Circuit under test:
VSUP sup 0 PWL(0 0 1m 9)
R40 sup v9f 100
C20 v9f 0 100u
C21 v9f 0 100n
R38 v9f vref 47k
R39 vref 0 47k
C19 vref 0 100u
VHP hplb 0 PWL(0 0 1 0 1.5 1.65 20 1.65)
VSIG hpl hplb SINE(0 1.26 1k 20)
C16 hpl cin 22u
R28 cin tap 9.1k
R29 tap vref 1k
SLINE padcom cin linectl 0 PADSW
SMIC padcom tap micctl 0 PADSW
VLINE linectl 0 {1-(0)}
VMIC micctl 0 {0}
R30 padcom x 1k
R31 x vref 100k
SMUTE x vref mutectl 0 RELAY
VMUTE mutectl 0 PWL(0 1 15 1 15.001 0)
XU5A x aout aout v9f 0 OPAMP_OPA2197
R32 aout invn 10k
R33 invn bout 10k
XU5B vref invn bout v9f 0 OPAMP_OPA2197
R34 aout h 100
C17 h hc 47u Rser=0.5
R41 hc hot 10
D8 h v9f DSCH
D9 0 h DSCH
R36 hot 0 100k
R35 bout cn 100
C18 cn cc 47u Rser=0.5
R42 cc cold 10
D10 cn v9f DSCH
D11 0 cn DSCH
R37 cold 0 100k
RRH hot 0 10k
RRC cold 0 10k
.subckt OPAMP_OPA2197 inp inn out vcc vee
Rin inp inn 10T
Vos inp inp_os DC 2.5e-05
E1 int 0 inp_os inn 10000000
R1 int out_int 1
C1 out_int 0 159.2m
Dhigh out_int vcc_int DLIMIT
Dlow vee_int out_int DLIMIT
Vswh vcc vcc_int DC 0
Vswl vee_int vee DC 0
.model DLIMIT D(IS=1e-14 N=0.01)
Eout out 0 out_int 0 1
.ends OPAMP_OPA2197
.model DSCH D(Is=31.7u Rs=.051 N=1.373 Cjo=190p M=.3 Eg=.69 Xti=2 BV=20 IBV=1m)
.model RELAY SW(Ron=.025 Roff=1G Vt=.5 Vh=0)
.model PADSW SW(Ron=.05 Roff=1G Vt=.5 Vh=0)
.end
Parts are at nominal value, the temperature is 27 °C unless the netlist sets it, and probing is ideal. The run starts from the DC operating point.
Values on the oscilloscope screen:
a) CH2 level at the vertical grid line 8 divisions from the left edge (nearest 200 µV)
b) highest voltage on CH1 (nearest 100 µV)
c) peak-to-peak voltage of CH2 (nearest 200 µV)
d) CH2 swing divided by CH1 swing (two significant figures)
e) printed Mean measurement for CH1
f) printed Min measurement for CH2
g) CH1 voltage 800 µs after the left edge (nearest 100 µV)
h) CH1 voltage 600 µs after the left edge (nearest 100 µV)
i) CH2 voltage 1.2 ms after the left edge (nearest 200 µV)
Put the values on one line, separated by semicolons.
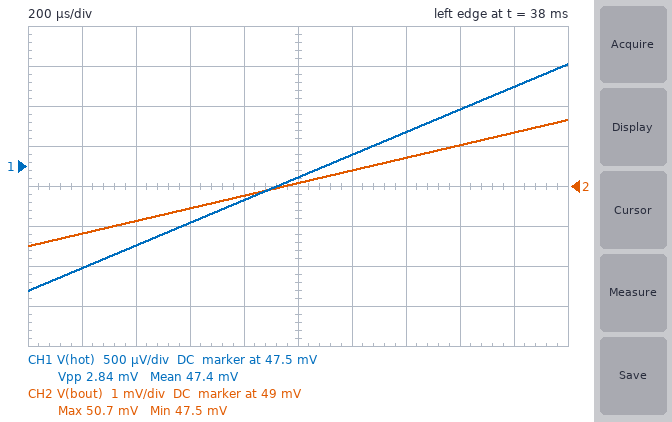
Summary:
50.0 mV; 48.8 mV; 3.2 mV; 1.1; 47.4 mV; 47.5 mV; 47.1 mV; 46.8 mV; 49.4 mV
